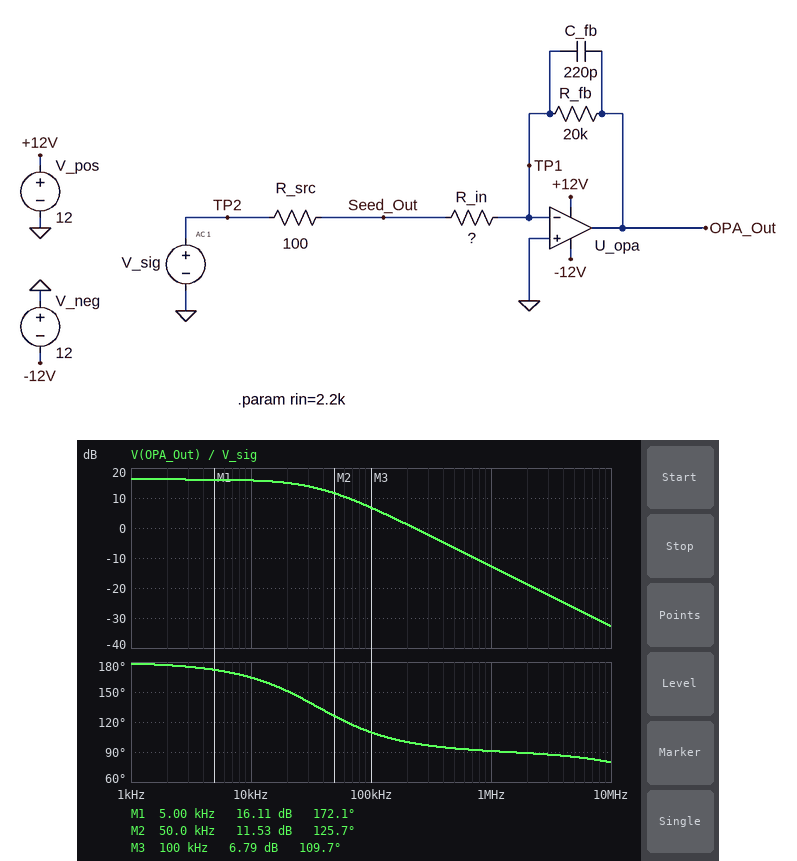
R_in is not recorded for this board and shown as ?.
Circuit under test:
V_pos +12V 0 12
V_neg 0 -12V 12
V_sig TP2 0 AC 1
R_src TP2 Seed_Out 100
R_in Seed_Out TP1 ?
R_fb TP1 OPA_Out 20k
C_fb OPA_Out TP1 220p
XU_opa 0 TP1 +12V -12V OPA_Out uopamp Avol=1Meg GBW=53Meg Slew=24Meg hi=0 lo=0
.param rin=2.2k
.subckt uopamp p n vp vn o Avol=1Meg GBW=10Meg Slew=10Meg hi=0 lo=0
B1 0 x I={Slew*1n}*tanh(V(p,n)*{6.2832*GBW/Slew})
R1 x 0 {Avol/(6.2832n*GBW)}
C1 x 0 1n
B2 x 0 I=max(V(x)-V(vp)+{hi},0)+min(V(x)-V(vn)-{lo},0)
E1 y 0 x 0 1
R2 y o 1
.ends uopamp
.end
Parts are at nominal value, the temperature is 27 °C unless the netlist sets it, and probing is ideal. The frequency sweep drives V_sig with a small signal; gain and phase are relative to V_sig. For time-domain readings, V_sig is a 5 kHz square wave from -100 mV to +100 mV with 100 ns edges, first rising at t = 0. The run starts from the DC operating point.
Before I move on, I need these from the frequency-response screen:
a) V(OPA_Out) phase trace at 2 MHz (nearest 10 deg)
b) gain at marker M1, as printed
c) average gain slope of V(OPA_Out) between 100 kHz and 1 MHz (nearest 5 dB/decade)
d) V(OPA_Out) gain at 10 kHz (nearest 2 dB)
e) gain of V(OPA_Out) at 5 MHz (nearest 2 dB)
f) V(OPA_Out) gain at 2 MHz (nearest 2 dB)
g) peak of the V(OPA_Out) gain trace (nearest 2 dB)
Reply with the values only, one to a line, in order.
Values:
90 deg
16.11 dB
-20 dB/decade
16 dB
-26 dB
-18 dB
16 dB
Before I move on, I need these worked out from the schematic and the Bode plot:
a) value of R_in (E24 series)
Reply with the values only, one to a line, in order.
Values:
3 kΩ
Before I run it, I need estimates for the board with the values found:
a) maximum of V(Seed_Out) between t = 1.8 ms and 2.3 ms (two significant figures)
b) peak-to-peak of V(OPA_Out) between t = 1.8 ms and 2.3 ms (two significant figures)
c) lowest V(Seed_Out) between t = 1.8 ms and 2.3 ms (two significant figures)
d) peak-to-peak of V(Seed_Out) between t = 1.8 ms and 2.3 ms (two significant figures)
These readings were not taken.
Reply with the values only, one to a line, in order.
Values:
97 mV
1.3 V
-97 mV
190 mV
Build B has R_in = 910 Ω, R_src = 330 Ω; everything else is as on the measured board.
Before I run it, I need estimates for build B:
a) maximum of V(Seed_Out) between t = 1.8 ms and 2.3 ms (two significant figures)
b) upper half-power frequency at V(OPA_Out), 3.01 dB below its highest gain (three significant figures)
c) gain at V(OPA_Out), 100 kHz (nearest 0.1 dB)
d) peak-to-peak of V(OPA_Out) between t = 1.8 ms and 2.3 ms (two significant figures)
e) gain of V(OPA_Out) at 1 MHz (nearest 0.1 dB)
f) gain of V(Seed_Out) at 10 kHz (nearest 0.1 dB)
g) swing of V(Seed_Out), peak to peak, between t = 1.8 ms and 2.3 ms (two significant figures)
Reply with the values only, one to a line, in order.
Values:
74 mV
35.8 kHz
14.7 dB
3.2 V
-4.8 dB
-2.7 dB
150 mV
